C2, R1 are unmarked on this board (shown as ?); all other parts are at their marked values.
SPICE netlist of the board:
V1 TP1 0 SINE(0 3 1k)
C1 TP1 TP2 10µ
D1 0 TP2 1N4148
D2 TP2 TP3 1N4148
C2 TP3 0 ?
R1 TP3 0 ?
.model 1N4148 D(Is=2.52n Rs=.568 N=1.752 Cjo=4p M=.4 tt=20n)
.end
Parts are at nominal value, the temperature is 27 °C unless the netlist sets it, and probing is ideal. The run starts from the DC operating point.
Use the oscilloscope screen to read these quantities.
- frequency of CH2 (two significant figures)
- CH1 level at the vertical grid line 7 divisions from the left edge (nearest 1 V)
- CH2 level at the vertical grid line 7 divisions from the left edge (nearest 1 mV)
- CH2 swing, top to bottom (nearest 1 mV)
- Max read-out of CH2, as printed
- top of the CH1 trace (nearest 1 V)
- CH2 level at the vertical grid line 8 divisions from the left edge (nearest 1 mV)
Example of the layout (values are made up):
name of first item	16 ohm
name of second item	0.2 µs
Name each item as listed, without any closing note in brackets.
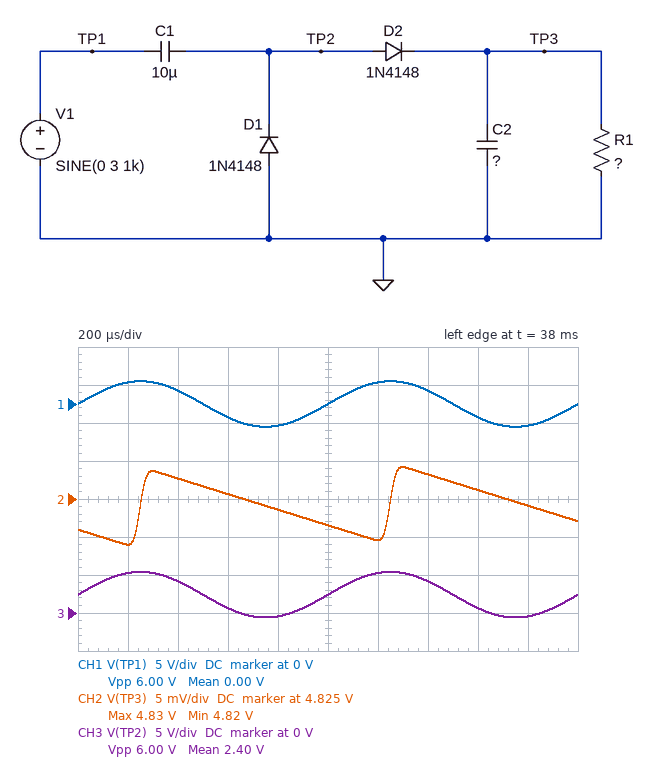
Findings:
frequency of CH2	1.0 kHz
CH1 level at the vertical grid line 7 divisions from the left edge	2 V
CH2 level at the vertical grid line 7 divisions from the left edge	4.828 V
CH2 swing, top to bottom	10 mV
Max read-out of CH2, as printed	4.83 V
top of the CH1 trace	3 V
CH2 level at the vertical grid line 8 divisions from the left edge	4.826 V
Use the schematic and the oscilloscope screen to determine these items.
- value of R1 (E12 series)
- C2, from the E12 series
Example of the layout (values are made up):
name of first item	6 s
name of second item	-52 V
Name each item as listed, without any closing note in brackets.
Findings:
value of R1	100 kΩ
C2, from the E12 series	4.7 µF
